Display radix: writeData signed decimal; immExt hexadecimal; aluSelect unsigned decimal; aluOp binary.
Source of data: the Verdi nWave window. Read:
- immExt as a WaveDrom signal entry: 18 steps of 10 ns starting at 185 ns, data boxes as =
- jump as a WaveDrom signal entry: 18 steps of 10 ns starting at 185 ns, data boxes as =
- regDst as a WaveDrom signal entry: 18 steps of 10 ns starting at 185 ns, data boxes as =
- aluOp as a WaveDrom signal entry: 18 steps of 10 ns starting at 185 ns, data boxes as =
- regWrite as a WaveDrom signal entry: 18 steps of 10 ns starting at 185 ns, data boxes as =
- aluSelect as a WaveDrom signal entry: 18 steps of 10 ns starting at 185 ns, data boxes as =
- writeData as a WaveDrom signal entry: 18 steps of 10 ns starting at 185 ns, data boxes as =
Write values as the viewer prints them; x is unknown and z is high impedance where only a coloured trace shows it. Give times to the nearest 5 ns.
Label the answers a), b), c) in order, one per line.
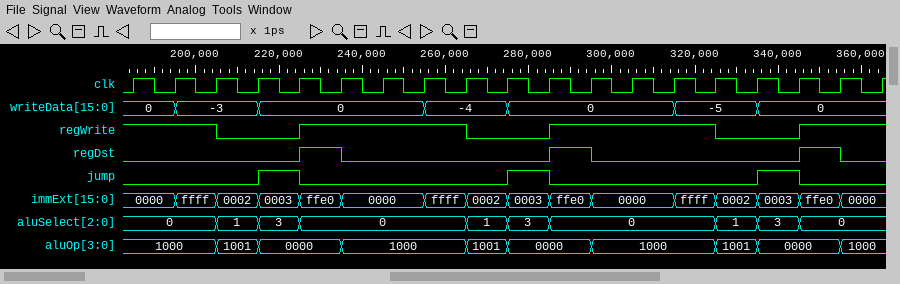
a) {name: 'immExt', wave: '======.=====.=====', data: '0000 ffff 0002 0003 ffe0 0000 ffff 0002 0003 ffe0 0000 ffff 0002 0003 ffe0 0000'}
b) {name: 'jump', wave: '0..10....10....10.'}
c) {name: 'regDst', wave: '0...10....10....10'}
d) {name: 'aluOp', wave: '=.==.=..==.=..==.=', data: '1000 1001 0000 1000 1001 0000 1000 1001 0000 1000'}
e) {name: 'regWrite', wave: '1.0.1...0.1...0.1.'}
f) {name: 'aluSelect', wave: '=.===...===...===.', data: '0 1 3 0 1 3 0 1 3 0'}
g) {name: 'writeData', wave: '==.=...=.=...=.=..', data: '0 -3 0 -4 0 -5 0'}
